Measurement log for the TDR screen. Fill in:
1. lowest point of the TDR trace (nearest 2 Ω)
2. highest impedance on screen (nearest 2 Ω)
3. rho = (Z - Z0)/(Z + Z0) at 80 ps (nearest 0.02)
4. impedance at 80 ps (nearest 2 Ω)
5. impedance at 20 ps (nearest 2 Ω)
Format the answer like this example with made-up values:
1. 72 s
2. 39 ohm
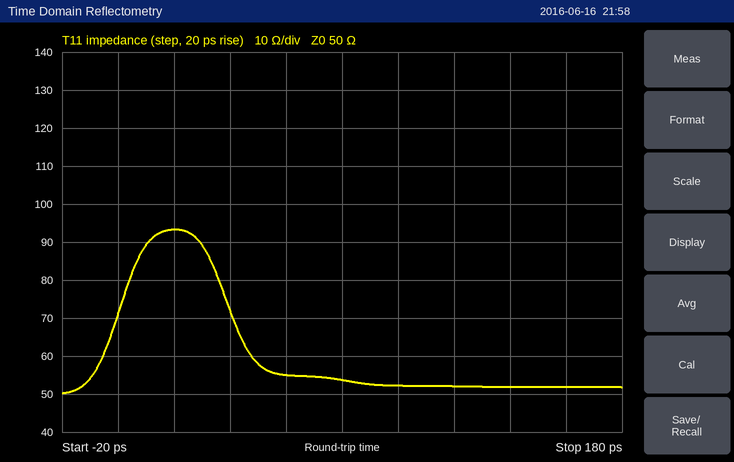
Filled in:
1. 50 Ω
2. 94 Ω
3. +0.04
4. 54 Ω
5. 94 Ω
